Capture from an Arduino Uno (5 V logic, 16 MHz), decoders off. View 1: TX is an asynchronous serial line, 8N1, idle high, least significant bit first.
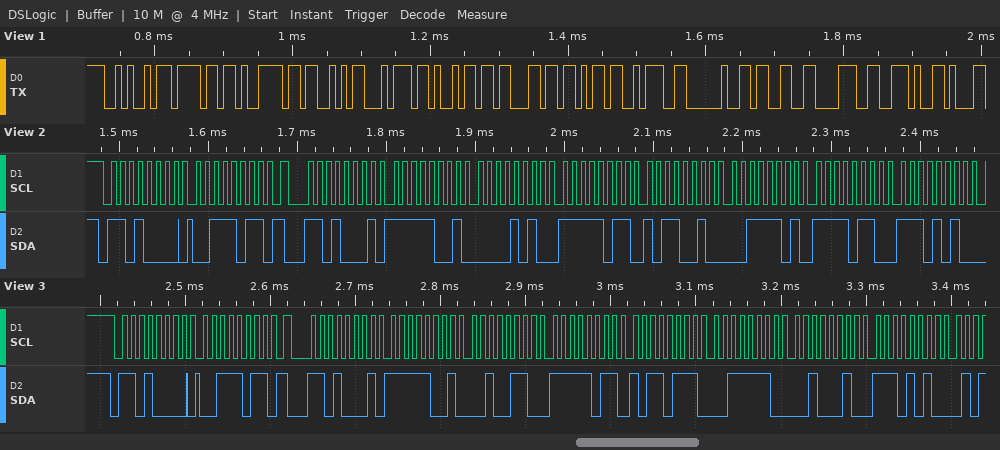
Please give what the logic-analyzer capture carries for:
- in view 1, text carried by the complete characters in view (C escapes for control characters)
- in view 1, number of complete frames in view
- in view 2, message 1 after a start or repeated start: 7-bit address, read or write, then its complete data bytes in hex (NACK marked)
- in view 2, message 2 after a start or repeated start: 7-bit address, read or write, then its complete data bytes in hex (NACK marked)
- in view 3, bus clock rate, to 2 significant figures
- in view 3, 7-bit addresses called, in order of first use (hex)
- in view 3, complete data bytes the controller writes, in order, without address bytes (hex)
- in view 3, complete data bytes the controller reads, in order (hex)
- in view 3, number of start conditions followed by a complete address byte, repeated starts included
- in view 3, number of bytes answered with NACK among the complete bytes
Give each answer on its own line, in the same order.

"JoyStick: 38."
13
0x68 write: 3B
0x68 read: F9 0A FB B2 3D F6 EA
100 kHz
0x68
3B
F9 26 FB B7 3E 22 EA
2
0
